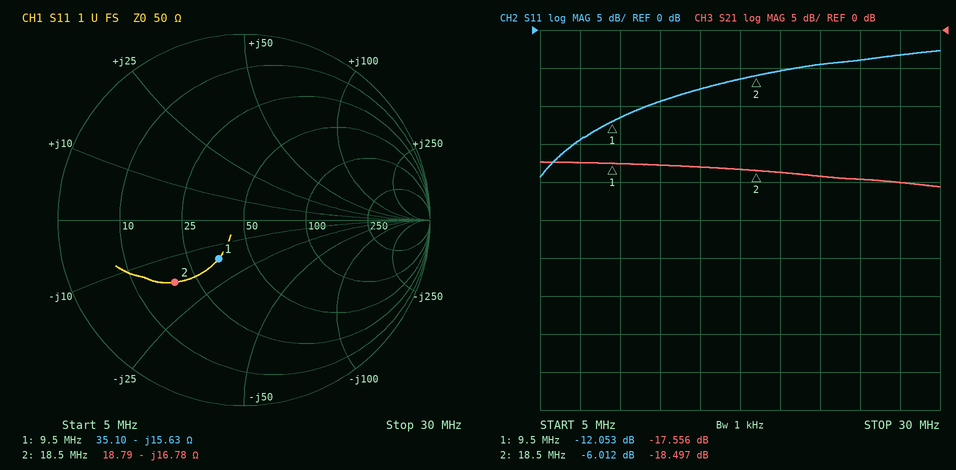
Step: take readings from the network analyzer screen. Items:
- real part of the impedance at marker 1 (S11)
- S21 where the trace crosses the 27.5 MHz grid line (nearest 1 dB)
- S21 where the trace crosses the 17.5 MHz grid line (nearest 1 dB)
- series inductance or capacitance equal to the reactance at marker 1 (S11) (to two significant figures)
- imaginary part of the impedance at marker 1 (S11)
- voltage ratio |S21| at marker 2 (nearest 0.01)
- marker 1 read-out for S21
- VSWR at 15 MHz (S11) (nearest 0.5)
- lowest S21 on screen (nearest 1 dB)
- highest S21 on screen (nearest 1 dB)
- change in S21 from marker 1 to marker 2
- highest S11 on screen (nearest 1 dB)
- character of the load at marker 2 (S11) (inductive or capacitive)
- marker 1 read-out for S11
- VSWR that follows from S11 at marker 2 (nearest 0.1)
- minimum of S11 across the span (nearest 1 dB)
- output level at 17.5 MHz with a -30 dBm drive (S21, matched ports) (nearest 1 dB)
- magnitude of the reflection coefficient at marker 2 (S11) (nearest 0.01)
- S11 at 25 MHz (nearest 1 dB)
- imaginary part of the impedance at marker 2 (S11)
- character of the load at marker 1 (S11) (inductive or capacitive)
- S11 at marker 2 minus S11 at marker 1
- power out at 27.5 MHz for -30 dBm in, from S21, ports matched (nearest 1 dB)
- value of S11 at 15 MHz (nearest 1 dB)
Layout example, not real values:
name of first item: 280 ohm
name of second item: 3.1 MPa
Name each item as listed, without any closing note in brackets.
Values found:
real part of the impedance at marker 1: 35.10 Ω
S21 where the trace crosses the 27.5 MHz grid line: -20 dB
S21 where the trace crosses the 17.5 MHz grid line: -18 dB
series inductance or capacitance equal to the reactance at marker 1 (S11): 1.1 nF
imaginary part of the impedance at marker 1: -15.63 Ω
voltage ratio |S21| at marker 2: 0.12
marker 1 read-out for S21: -17.556 dB
VSWR at 15 MHz (S11): 2.5
lowest S21 on screen: -21 dB
highest S21 on screen: -17 dB
change in S21 from marker 1 to marker 2: -0.941 dB
highest S11 on screen: -3 dB
character of the load at marker 2 (S11): capacitive
marker 1 read-out for S11: -12.053 dB
VSWR that follows from S11 at marker 2: 3.0
minimum of S11 across the span: -19 dB
output level at 17.5 MHz with a -30 dBm drive (S21, matched ports): -48 dBm
magnitude of the reflection coefficient at marker 2 (S11): 0.50
S11 at 25 MHz: -4 dB
imaginary part of the impedance at marker 2: -16.78 Ω
character of the load at marker 1 (S11): capacitive
S11 at marker 2 minus S11 at marker 1: 6.041 dB
power out at 27.5 MHz for -30 dBm in, from S21, ports matched: -50 dBm
value of S11 at 15 MHz: -8 dB
